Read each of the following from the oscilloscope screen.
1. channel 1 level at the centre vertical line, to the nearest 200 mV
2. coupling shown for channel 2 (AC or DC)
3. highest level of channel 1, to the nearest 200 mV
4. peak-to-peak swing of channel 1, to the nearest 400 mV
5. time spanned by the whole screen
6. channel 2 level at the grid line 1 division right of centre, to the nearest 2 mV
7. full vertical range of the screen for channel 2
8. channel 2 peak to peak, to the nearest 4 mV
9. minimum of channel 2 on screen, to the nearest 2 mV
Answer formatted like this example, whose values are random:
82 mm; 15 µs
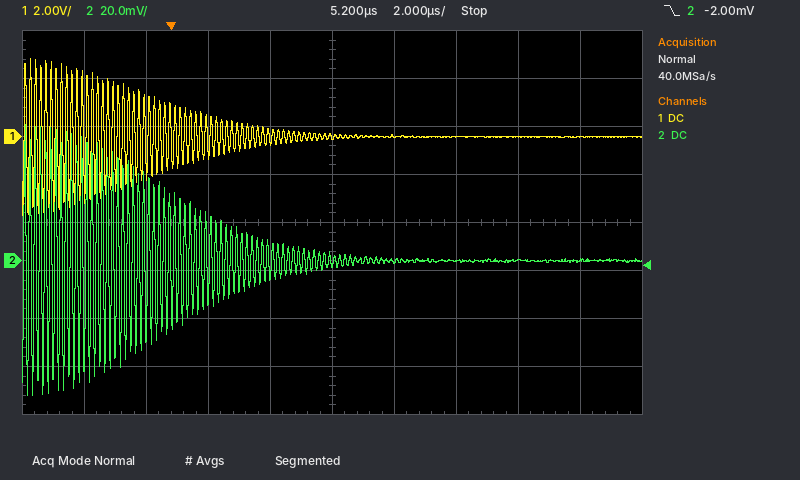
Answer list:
0.0 V; DC; 3.2 V; 6.4 V; 20 µs; 0 mV; 160 mV; 112 mV; -56 mV
